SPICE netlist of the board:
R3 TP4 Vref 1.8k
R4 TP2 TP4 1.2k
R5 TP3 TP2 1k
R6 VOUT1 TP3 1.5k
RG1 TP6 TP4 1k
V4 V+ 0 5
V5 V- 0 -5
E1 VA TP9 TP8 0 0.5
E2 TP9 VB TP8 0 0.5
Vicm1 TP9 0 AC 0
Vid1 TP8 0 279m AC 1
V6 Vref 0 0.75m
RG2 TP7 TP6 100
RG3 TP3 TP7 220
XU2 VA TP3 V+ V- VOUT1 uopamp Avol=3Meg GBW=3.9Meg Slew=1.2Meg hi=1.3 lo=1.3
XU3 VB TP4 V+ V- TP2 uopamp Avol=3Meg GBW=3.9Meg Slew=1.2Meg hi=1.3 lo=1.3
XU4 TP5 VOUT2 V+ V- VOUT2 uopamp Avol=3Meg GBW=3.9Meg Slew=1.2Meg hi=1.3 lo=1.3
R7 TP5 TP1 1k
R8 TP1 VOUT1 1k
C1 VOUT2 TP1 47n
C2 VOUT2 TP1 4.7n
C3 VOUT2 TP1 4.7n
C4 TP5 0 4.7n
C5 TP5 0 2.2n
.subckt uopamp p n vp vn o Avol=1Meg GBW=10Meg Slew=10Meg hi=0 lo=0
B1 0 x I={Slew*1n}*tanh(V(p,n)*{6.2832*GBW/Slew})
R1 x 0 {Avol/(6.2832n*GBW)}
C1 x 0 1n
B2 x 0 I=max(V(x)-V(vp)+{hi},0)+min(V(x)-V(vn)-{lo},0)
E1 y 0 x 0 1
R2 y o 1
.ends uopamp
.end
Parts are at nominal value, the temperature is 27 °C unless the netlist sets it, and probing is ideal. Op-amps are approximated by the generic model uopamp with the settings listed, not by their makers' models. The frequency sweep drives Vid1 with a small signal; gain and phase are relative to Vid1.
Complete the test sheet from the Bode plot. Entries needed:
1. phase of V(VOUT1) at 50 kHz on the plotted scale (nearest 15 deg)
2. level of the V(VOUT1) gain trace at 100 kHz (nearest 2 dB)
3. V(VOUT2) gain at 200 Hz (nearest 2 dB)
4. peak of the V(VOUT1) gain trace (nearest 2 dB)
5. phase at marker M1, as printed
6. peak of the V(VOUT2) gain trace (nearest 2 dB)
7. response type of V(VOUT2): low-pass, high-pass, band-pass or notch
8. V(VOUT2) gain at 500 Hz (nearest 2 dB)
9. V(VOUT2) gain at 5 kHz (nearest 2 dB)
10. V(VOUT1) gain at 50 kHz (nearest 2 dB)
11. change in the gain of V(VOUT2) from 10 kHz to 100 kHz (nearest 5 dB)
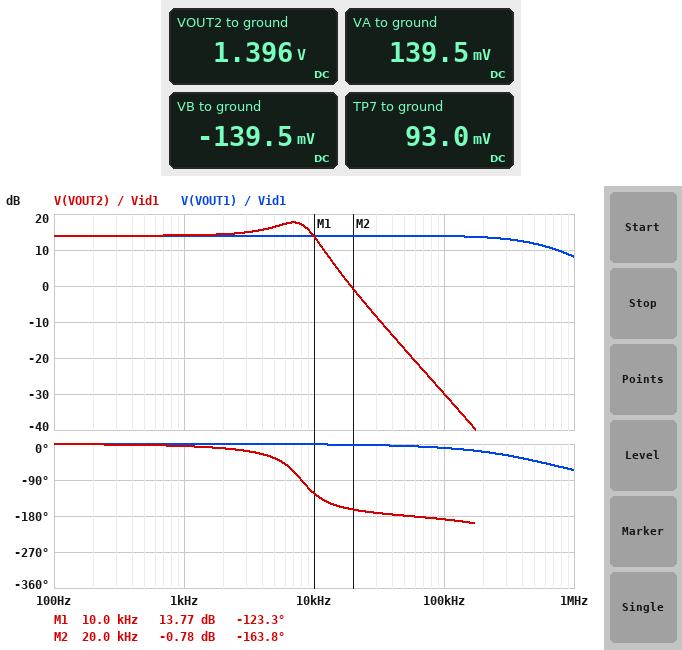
0 deg
14 dB
14 dB
14 dB
-123.3 deg
18 dB
low-pass
14 dB
16 dB
14 dB
-45 dB
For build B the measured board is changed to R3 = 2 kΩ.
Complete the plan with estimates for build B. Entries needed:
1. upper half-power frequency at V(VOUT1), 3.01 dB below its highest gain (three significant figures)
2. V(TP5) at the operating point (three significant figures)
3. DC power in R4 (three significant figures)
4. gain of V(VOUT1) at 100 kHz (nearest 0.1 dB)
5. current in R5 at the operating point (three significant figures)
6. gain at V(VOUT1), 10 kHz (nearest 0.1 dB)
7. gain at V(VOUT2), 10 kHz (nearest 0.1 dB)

612 kHz
1.38 V
95.1 µW
13.8 dB
617 µA
13.9 dB
13.7 dB
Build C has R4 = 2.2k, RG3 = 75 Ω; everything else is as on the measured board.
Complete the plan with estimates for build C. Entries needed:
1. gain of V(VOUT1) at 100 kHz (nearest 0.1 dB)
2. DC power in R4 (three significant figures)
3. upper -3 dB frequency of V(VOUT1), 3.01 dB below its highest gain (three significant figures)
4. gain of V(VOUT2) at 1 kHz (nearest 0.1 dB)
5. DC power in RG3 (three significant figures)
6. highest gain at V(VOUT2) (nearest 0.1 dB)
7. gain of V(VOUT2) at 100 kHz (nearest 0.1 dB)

16.7 dB
219 µW
415 kHz
17.0 dB
4.23 µW
20.6 dB
-27.1 dB
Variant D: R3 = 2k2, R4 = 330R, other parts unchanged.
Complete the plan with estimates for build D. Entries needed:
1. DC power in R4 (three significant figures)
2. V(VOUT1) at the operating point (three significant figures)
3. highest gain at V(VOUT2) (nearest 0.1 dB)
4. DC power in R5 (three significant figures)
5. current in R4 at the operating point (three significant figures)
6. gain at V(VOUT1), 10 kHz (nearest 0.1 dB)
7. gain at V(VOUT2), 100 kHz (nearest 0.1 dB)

25.0 µW
1.01 V
14.9 dB
137 µW
275 µA
11.2 dB
-32.6 dB
